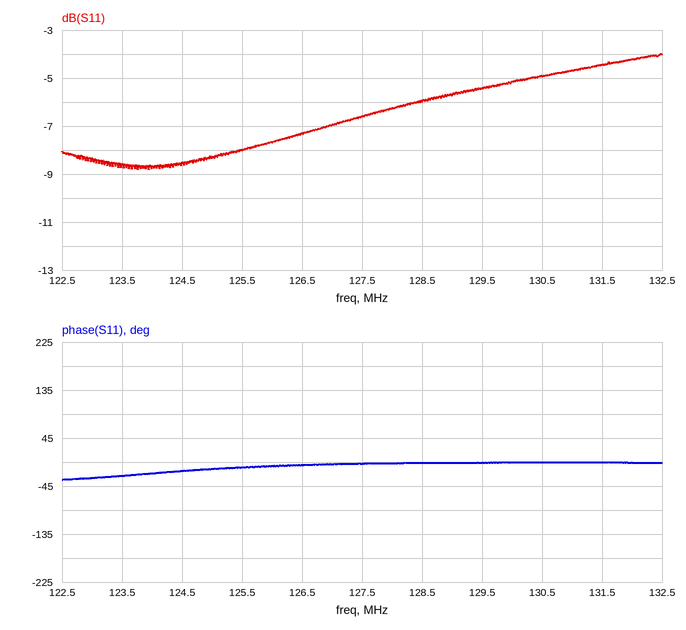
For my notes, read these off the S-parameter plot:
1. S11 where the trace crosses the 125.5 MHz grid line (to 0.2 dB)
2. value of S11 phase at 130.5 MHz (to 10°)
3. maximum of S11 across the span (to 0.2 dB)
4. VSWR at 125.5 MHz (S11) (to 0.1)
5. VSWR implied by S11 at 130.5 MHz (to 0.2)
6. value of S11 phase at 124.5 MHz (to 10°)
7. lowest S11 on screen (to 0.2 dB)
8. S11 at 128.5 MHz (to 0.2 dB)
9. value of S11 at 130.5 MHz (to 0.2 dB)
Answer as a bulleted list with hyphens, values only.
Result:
- -8.0 dB
- 0°
- -4.0 dB
- 2.3
- 3.6
- -20°
- -8.8 dB
- -6.0 dB
- -5.0 dB
